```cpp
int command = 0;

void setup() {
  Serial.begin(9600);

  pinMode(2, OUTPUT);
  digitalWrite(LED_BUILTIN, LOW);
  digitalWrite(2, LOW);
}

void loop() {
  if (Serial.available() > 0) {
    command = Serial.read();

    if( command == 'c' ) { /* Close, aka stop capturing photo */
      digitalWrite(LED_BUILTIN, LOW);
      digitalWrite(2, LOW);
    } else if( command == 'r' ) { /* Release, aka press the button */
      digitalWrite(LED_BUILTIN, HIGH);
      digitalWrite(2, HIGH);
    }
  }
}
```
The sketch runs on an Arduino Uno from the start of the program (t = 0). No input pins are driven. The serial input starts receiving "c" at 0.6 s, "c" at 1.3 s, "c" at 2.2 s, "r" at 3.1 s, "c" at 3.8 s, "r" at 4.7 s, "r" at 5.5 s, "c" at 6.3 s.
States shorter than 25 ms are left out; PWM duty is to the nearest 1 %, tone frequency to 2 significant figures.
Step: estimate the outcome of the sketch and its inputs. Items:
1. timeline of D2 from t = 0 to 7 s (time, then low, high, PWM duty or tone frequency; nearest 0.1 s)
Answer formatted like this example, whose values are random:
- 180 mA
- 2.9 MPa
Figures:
- 0 s low; 3.1 s high; 3.8 s low; 4.7 s high; 6.3 s low
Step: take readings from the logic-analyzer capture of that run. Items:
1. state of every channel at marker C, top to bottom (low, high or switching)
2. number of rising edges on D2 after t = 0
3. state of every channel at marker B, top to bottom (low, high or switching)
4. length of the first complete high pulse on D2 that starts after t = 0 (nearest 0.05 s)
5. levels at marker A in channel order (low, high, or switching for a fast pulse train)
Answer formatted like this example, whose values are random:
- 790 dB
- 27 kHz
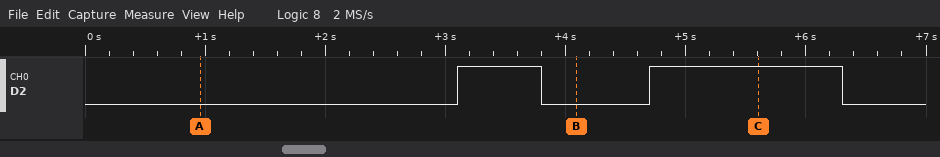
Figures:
- D2 high
- 2
- D2 low
- 0.70 s
- D2 low
